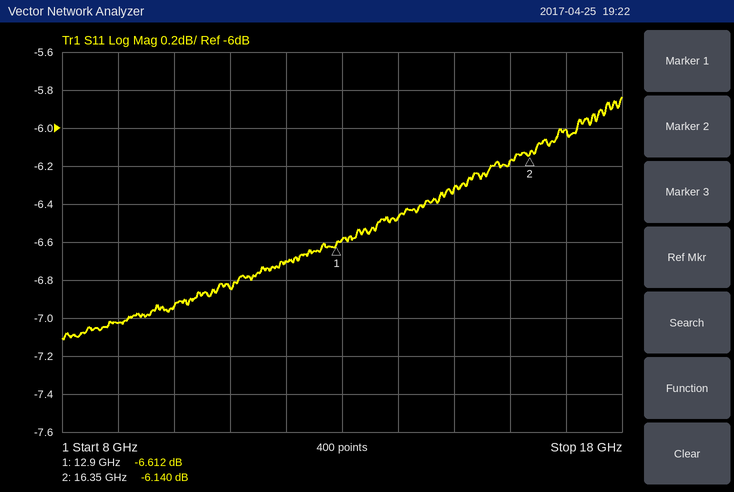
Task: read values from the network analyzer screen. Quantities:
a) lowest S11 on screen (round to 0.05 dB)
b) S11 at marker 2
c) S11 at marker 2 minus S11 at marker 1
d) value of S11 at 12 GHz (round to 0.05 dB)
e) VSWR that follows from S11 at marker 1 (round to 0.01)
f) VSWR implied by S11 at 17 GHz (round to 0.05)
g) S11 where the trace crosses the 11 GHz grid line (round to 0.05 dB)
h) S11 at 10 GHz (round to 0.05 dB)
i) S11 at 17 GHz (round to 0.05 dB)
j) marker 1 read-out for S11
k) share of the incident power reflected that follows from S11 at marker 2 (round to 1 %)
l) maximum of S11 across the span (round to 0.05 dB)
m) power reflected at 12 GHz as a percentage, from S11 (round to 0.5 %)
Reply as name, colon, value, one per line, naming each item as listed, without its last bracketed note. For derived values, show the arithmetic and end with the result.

lowest S11 on screen: -7.10 dB
S11 at marker 2: -6.140 dB
S11 at marker 2 minus S11 at marker 1: -6.14 − (-6.612) = 0.472 dB
value of S11 at 12 GHz: -6.70 dB
VSWR that follows from S11 at marker 1: (1 + 0.4671)/(1 − 0.4671) ≈ 2.75
VSWR implied by S11 at 17 GHz: |Γ| = 10^(-6/20) = 0.5012; VSWR = (1 + 0.5012)/(1 − 0.5012) ≈ 3.01, so 3.00 to the nearest 0.05
S11 where the trace crosses the 11 GHz grid line: -6.85 dB
S11 at 10 GHz: -6.95 dB
S11 at 17 GHz: -6.00 dB
marker 1 read-out for S11: -6.612 dB
share of the incident power reflected that follows from S11 at marker 2: 10^(-6.14/10) ≈ 24 %
maximum of S11 across the span: -5.85 dB
power reflected at 12 GHz as a percentage, from S11: 10^(-6.7/10) ≈ 21.4 %, so 21.5 % to the nearest 0.5 %
